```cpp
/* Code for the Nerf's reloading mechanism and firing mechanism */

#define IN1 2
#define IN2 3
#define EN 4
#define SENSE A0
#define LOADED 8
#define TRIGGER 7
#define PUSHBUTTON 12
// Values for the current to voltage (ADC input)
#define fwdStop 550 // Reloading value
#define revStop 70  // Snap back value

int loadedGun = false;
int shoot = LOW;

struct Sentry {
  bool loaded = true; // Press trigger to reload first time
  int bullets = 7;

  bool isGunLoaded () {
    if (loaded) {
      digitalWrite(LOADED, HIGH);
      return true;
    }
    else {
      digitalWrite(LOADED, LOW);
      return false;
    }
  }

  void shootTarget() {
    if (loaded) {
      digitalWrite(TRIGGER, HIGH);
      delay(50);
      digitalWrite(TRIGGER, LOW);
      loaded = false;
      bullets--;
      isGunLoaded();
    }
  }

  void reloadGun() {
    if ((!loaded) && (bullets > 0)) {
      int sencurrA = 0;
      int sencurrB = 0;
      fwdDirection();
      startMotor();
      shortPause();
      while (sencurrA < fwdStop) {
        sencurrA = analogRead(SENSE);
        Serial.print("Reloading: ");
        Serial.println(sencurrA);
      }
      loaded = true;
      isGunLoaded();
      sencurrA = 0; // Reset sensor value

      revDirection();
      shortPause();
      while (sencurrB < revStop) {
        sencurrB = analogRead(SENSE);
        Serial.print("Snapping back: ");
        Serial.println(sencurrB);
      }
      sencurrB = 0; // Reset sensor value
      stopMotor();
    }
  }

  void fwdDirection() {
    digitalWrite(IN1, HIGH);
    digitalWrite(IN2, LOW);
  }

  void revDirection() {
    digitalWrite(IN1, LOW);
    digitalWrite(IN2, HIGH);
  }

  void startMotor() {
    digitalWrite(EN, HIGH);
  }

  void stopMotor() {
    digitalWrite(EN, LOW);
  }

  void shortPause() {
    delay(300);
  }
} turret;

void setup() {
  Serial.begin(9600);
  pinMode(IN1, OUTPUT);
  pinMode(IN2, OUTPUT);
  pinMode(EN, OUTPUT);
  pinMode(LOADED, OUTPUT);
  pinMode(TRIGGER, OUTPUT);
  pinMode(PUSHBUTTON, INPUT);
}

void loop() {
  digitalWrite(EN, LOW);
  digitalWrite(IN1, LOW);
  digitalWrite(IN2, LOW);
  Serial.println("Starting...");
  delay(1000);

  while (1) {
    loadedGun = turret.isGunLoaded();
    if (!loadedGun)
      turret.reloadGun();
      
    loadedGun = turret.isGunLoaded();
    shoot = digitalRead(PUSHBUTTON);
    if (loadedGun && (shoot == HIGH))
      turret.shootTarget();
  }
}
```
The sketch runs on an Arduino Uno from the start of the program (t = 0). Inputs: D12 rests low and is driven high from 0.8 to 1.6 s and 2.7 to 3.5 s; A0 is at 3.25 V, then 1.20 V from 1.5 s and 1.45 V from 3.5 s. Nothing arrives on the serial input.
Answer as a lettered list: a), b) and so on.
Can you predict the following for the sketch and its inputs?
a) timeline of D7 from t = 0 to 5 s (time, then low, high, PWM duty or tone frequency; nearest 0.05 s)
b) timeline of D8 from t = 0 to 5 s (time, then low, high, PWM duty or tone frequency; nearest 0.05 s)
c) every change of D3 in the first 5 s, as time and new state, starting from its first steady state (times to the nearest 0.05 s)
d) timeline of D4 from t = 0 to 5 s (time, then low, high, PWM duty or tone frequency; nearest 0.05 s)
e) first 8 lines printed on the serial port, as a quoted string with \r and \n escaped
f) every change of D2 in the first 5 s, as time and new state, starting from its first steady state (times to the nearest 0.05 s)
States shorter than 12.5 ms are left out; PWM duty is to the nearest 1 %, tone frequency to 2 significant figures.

a) 0 s low; 1 s high; 1.05 s low; 2.7 s high; 2.75 s low
b) 0 s low; 1 s high; 1.05 s low; 1.35 s high; 2.75 s low
c) 0 s low; 1.35 s high; 2.75 s low
d) 0 s low; 1.05 s high; 1.65 s low; 2.75 s high
e) "Starting...\r\nReloading: 665\r\nSnapping back: 245\r\nReloading: 245\r\nReloading: 245\r\nReloading: 245\r\nReloading: 245\r\nReloading: 245\r\n"
f) 0 s low; 1.05 s high; 1.35 s low; 2.75 s high
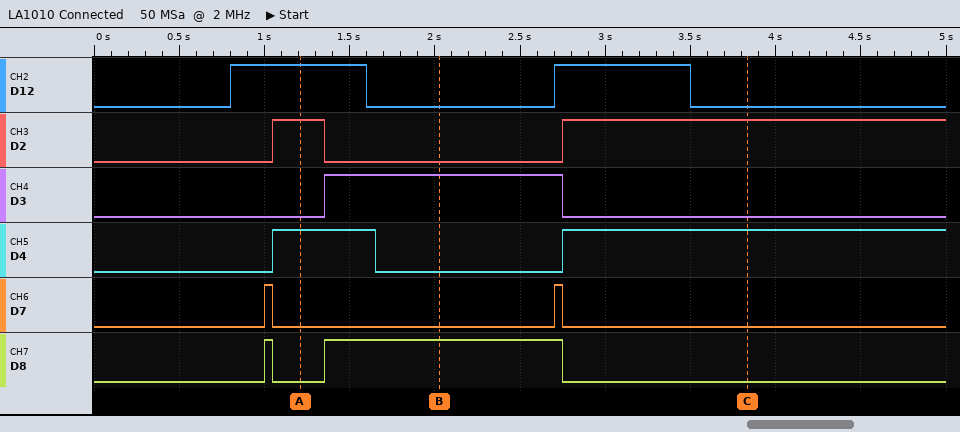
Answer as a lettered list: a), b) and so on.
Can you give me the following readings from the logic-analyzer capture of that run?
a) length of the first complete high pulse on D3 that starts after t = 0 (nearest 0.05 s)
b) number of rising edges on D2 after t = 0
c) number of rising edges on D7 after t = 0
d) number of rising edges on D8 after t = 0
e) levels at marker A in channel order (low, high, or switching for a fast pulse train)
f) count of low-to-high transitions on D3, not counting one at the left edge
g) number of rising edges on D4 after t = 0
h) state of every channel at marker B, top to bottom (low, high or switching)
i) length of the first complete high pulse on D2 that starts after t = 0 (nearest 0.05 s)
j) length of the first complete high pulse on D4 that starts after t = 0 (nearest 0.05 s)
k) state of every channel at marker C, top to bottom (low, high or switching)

a) 1.40 s
b) 2
c) 2
d) 2
e) D12 high, D2 high, D3 low, D4 high, D7 low, D8 low
f) 1
g) 2
h) D12 low, D2 low, D3 high, D4 low, D7 low, D8 high
i) 0.30 s
j) 0.60 s
k) D12 low, D2 high, D3 low, D4 high, D7 low, D8 low
